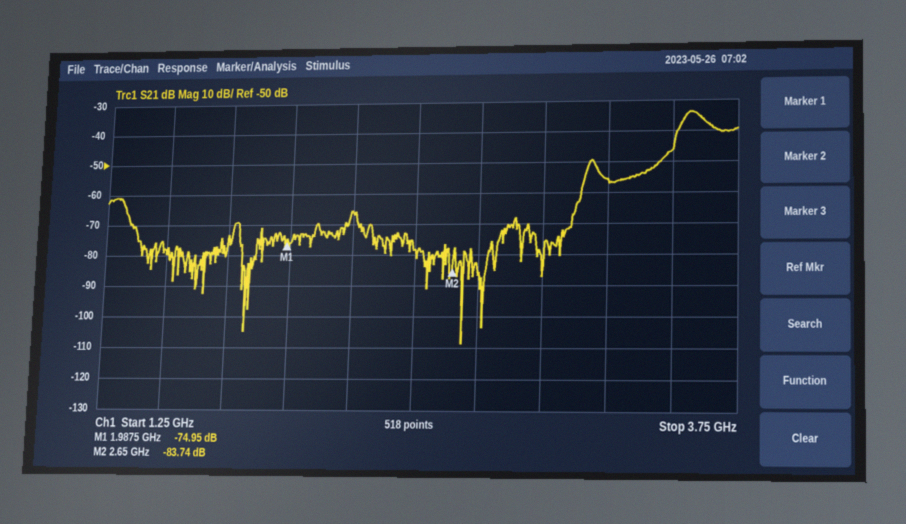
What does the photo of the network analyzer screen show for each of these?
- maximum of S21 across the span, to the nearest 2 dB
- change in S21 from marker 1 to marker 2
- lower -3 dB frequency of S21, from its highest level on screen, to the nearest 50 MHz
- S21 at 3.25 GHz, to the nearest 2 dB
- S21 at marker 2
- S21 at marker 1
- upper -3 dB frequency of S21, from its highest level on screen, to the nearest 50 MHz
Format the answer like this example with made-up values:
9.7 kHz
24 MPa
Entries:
-34 dB
-8.79 dB
3.55 GHz
-56 dB
-83.74 dB
-74.95 dB
3.60 GHz
